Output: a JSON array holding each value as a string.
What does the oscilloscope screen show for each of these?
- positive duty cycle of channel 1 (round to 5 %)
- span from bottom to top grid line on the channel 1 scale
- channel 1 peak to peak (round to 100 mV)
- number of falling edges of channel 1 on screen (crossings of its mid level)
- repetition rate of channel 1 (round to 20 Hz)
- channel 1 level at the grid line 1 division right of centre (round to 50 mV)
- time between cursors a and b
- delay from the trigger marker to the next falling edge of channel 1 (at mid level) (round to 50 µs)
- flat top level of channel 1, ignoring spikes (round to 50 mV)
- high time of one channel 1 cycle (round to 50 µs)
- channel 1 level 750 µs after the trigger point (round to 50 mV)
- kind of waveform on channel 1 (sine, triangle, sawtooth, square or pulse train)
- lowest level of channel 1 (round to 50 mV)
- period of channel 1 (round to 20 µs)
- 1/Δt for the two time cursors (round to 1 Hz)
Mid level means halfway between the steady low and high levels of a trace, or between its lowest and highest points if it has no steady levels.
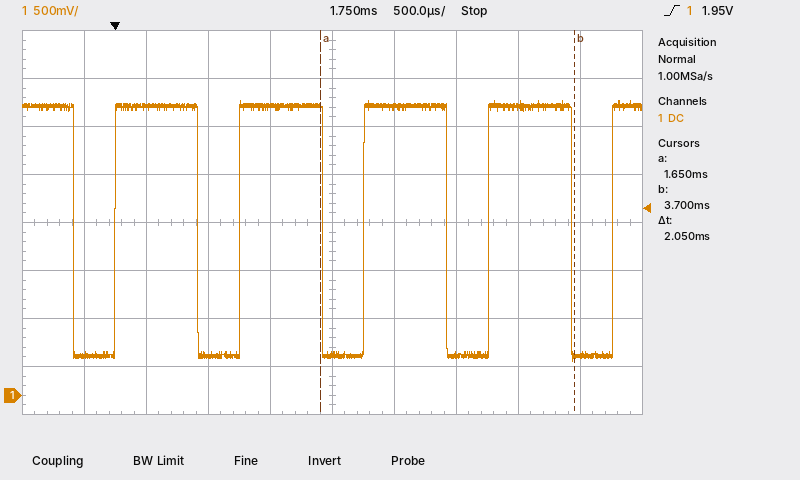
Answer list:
["65 %", "4 V", "2.70 V", "5", "1.00 kHz", "3.00 V", "2.05 ms", "650 µs", "3.00 V", "650 µs", "400 mV", "pulse train", "350 mV", "1.00 ms", "488 Hz"]
